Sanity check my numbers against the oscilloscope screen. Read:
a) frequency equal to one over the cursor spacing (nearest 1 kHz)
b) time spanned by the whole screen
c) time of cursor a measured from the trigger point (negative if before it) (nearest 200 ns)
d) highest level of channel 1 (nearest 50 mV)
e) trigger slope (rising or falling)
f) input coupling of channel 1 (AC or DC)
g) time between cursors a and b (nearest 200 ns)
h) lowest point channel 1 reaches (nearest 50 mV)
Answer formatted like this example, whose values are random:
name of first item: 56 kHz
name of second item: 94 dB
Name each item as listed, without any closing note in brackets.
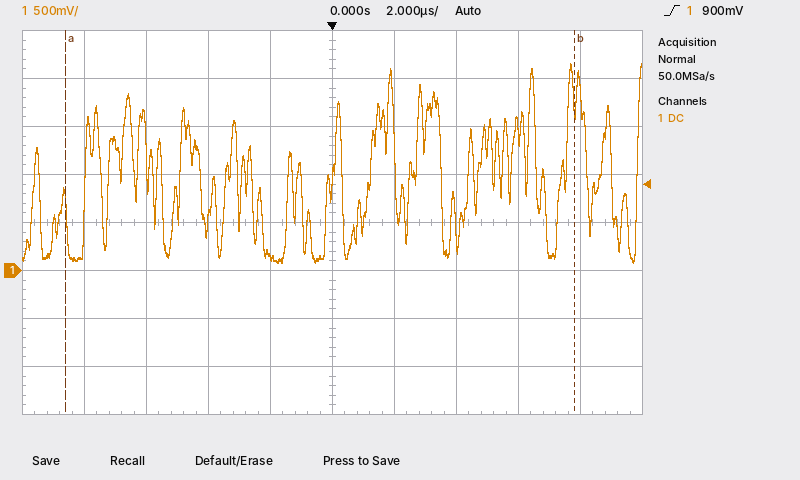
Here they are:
frequency equal to one over the cursor spacing: 61 kHz
time spanned by the whole screen: 20 µs
time of cursor a measured from the trigger point (negative if before it): -8.6 µs
highest level of channel 1: 2.15 V
trigger slope: rising
input coupling of channel 1: DC
time between cursors a and b: 16.4 µs
lowest point channel 1 reaches: 100 mV
